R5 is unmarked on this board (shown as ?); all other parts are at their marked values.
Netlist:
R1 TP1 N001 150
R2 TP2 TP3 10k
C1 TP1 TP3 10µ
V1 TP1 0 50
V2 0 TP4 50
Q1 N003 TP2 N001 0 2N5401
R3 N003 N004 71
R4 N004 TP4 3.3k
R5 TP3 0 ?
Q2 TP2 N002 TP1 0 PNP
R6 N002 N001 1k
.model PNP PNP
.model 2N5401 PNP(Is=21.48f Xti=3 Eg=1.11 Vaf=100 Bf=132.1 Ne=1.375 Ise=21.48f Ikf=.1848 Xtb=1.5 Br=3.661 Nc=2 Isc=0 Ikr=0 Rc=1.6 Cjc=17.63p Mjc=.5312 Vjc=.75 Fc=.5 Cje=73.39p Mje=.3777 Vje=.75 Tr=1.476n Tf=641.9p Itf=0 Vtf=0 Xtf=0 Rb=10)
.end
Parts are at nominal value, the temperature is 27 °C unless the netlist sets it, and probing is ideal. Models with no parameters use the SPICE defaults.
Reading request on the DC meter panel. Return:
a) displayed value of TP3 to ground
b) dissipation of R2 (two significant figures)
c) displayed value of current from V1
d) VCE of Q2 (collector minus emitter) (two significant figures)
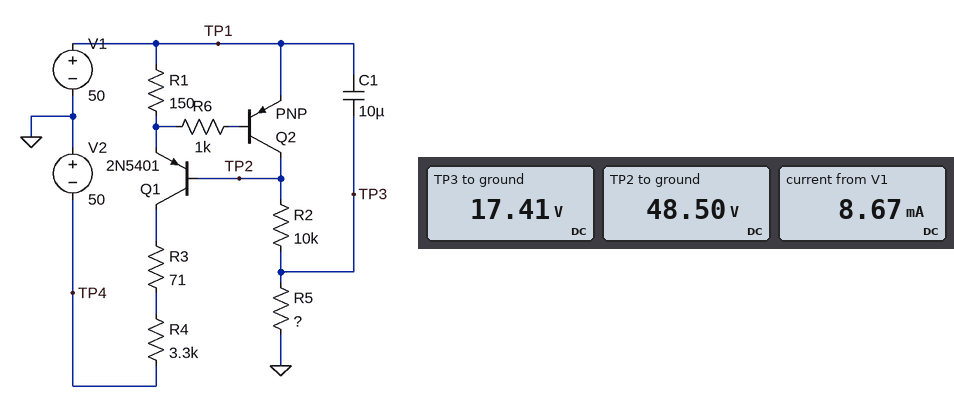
17.41 V
97 mW
8.67 mA
-1.5 V
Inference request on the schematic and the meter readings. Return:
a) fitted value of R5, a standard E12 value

5.6 kΩ
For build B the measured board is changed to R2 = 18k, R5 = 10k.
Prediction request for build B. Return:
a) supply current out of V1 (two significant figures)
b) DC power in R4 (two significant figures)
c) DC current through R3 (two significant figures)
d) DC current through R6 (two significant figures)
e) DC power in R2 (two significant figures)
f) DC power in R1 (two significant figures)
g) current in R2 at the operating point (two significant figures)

7.1 mA
95 mW
5.4 mA
17 µA
54 mW
4.3 mW
1.7 mA
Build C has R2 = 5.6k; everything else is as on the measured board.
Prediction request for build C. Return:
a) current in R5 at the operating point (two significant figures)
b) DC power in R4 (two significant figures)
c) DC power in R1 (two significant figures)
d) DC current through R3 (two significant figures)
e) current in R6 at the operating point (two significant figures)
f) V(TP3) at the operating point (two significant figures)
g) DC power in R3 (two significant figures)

4.3 mA
110 mW
4.9 mW
5.7 mA
43 µA
24 V
2.3 mW
